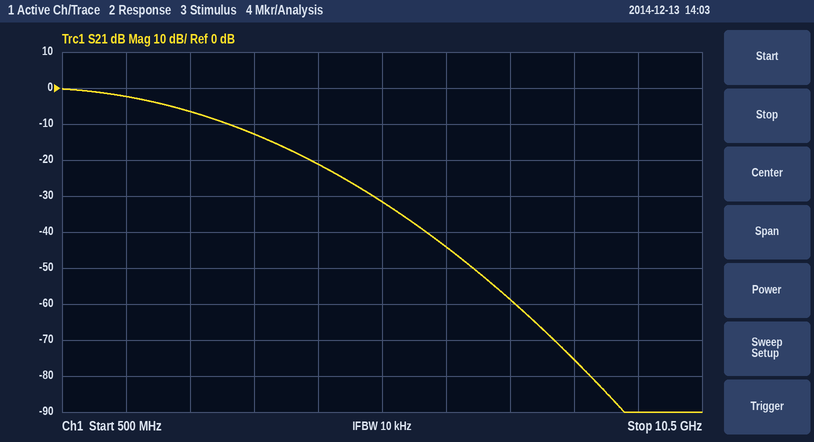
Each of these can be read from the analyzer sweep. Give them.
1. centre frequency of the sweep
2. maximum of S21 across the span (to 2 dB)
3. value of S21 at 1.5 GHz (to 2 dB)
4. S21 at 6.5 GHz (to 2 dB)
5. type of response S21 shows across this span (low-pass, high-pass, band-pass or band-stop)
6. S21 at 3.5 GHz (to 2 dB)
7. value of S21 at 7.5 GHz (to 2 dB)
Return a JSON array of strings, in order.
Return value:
["5.5 GHz", "0 dB", "-2 dB", "-44 dB", "low-pass", "-12 dB", "-58 dB"]
